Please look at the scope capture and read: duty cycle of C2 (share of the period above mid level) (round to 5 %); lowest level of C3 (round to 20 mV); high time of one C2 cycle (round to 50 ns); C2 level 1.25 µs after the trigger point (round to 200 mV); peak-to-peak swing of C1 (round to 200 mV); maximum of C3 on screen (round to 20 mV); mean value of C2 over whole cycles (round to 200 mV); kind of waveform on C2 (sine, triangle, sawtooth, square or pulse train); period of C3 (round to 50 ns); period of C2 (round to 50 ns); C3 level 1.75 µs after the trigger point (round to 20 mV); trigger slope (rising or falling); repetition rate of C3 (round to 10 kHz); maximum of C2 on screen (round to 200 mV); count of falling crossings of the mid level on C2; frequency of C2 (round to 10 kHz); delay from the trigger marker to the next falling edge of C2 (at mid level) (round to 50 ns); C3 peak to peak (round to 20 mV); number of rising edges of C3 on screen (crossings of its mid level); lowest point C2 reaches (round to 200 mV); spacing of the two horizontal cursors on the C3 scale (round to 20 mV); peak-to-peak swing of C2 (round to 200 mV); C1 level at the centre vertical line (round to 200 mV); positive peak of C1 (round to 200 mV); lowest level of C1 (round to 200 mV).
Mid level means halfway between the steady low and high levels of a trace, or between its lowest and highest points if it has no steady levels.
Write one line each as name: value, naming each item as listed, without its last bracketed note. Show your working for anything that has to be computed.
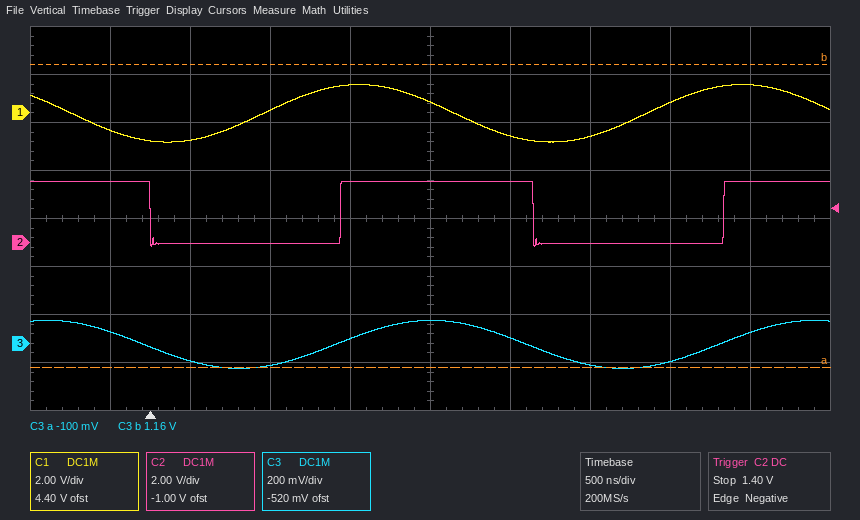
duty cycle of C2 (share of the period above mid level): 1.20 µs / 2.40 µs ≈ 50 %
lowest level of C3: -100 mV
high time of one C2 cycle: 1.20 µs
C2 level 1.25 µs after the trigger point: 2.6 V
peak-to-peak swing of C1: 1.2 V − (-1.2 V) = 2.4 V
maximum of C3 on screen: 100 mV
mean value of C2 over whole cycles: -200 mV + 0.5 × (2.6 V − (-200 mV)) ≈ 1.2 V
kind of waveform on C2: square
period of C3: 2.40 µs
period of C2: 2.40 µs
C3 level 1.75 µs after the trigger point: 100 mV
trigger slope: falling
repetition rate of C3: 1 / 2.40 µs ≈ 417 kHz, so 420 kHz to the nearest 10 kHz
maximum of C2 on screen: 2.6 V
count of falling crossings of the mid level on C2: 2
frequency of C2: 1 / 2.40 µs ≈ 417 kHz, so 420 kHz to the nearest 10 kHz
delay from the trigger marker to the next falling edge of C2 (at mid level): 2.40 µs
C3 peak to peak: 100 mV − (-100 mV) = 200 mV
number of rising edges of C3 on screen: 2
lowest point C2 reaches: -200 mV
spacing of the two horizontal cursors on the C3 scale: 1.26 V
peak-to-peak swing of C2: 2.6 V − (-200 mV) = 2.8 V
C1 level at the centre vertical line: 400 mV
positive peak of C1: 1.2 V
lowest level of C1: -1.2 V
